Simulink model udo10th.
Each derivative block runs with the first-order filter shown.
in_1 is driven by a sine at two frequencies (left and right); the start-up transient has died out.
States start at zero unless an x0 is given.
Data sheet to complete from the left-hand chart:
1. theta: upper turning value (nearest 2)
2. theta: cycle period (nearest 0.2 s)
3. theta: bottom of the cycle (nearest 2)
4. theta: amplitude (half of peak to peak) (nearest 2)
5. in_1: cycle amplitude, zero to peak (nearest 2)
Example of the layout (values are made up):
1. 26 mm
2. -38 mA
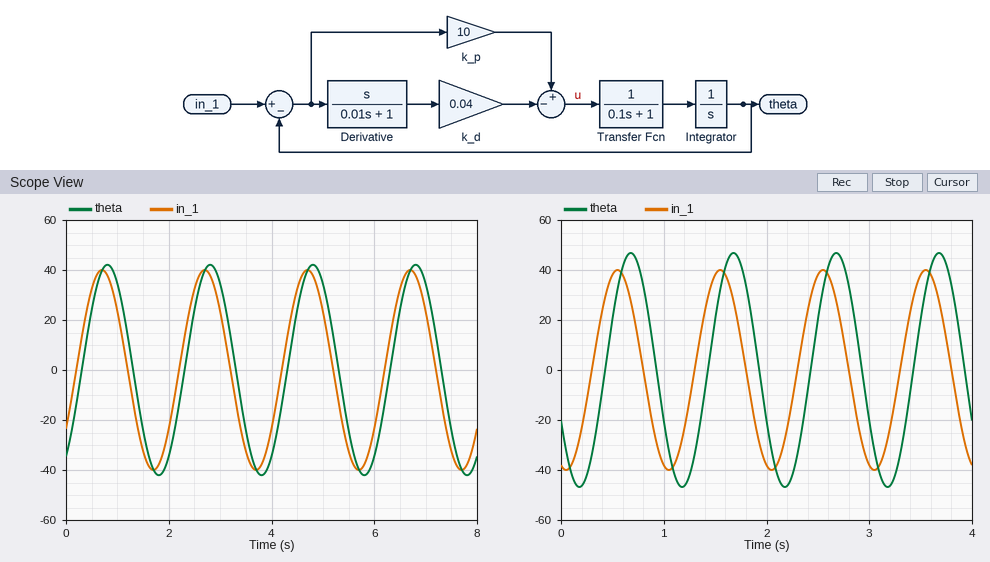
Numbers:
1. 42
2. 2.0 s
3. -42
4. 42
5. 40
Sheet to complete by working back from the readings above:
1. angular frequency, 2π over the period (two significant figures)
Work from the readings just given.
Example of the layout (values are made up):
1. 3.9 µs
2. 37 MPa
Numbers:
1. 3.1 rad/s
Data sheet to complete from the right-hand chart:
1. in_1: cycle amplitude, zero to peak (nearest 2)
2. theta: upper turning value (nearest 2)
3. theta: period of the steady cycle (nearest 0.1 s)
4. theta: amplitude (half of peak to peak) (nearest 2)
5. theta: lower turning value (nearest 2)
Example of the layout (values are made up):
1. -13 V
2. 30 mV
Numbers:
1. 40
2. 46
3. 1.0 s
4. 46
5. -46
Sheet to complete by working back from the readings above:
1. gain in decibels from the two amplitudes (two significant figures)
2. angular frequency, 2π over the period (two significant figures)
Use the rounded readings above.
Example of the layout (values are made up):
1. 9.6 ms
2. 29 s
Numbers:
1. 1.2 dB
2. 6.3 rad/s
